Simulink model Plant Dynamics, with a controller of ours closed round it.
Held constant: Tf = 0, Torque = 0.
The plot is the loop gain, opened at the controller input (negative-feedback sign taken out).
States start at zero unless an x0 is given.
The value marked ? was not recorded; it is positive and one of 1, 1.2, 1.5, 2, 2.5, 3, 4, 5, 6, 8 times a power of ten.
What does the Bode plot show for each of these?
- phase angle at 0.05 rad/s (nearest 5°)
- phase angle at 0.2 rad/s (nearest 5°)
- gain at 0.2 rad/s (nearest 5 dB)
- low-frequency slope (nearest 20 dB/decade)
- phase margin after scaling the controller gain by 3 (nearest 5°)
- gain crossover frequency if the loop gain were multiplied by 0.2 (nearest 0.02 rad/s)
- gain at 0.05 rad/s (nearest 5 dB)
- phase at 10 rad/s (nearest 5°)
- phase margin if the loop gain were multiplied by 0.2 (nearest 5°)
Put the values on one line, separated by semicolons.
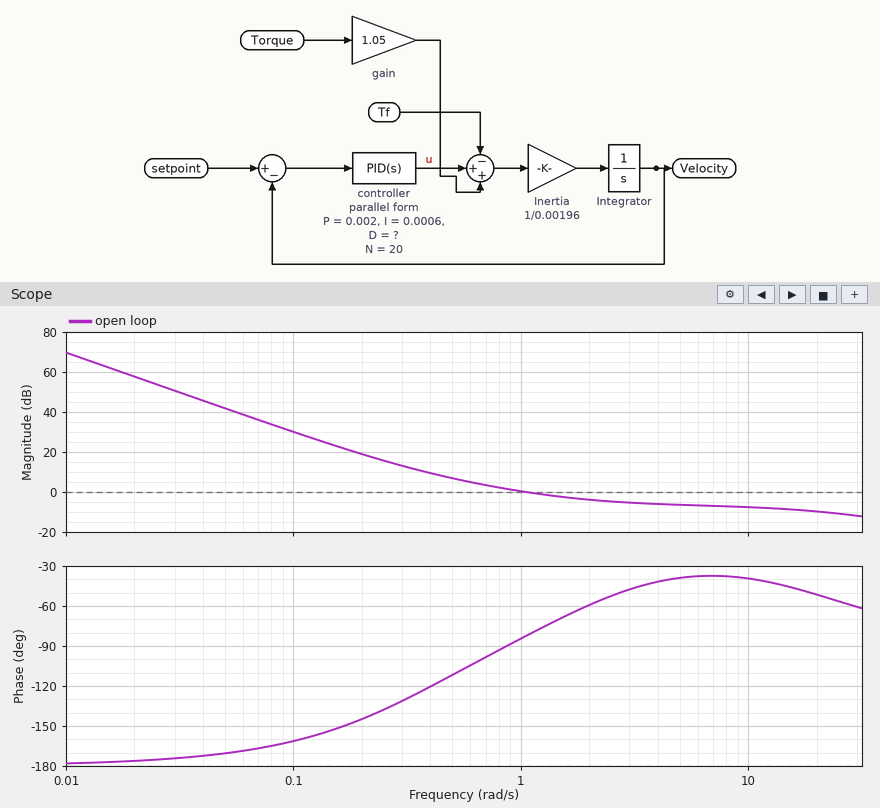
-170°; -145°; 20 dB; -40 dB/decade; 130°; 0.28 rad/s; 40 dB; -40°; 45°
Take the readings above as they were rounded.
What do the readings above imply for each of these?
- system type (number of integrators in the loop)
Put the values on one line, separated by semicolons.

2
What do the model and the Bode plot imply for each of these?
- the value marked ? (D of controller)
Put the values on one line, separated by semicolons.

0.0008
